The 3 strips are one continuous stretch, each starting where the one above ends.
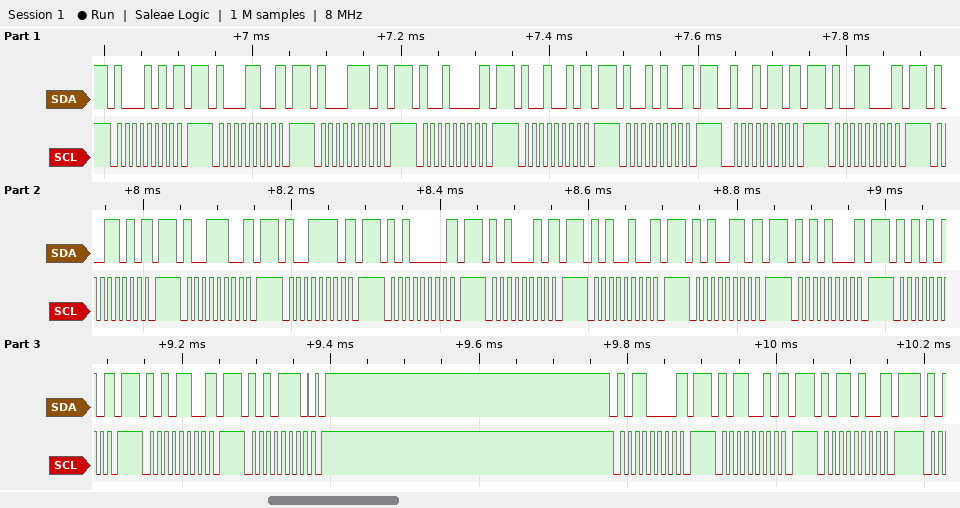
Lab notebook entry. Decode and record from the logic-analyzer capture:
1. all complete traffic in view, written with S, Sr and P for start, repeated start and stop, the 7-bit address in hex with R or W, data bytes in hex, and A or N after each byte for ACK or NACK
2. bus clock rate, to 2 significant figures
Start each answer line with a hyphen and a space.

- S 45W N P S 46W N P S 47W N P S 48W N P S 49W N P S 4AW N P S 4BW N P S 4CW N P S 4DW N P S 4EW N P S 4FW N P S 50W N P S 51W N P S 52W N P S 53W N P S 54W N P S 55W N P S 56W N P S 57W A P S 58W N P S 59W N P S 5AW N P
- 100 kHz
